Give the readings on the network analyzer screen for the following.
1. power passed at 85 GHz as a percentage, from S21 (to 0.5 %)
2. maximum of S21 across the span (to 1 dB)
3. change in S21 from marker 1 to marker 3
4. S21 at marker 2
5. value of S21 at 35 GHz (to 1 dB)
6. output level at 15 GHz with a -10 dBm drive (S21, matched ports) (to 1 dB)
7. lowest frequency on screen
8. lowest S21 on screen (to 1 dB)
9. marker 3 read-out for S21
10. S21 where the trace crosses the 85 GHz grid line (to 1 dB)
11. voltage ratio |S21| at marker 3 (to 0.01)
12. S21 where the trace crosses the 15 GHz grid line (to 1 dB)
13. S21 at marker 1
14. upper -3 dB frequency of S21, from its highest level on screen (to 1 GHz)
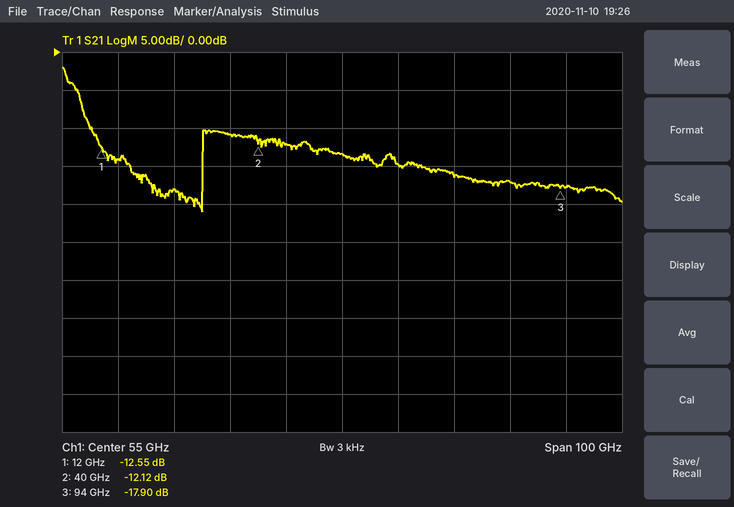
2.0 %
-2 dB
-5.35 dB
-12.12 dB
-11 dB
-24 dBm
5 GHz
-21 dB
-17.90 dB
-17 dB
0.13
-14 dB
-12.55 dB
8 GHz
